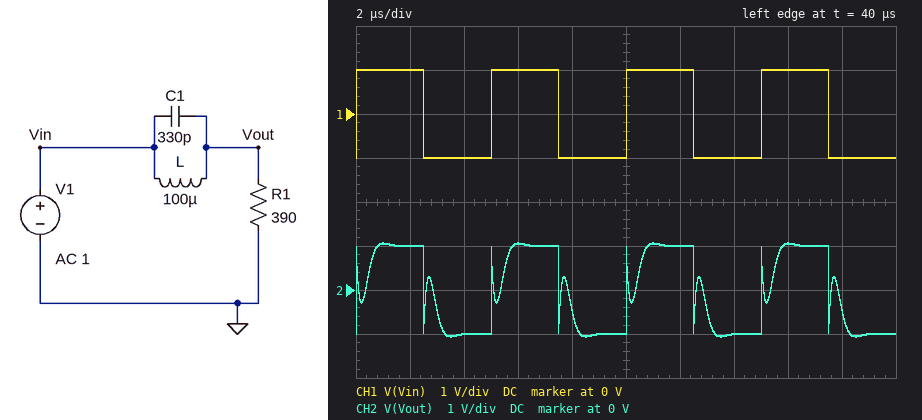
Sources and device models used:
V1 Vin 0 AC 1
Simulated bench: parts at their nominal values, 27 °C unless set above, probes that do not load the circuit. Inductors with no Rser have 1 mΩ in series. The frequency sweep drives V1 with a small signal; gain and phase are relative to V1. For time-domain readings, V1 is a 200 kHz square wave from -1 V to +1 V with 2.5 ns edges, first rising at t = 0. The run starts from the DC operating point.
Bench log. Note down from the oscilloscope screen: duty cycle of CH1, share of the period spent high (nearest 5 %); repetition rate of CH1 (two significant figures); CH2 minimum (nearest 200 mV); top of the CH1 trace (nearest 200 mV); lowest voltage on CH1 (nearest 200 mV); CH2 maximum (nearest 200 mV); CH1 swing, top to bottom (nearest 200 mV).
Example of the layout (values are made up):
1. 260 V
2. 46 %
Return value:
1. 50 %
2. 200 kHz
3. -1.0 V
4. 1.0 V
5. -1.0 V
6. 1.0 V
7. 2.0 V
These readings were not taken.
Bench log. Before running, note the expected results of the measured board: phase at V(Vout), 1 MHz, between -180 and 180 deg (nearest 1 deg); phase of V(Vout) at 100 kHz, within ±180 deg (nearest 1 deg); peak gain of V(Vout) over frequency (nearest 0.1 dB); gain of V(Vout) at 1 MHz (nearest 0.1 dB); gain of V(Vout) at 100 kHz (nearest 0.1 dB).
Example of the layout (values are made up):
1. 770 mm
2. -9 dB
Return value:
1. 79 deg
2. -9 deg
3. 0 dB
4. -14.7 dB
5. -0.1 dB
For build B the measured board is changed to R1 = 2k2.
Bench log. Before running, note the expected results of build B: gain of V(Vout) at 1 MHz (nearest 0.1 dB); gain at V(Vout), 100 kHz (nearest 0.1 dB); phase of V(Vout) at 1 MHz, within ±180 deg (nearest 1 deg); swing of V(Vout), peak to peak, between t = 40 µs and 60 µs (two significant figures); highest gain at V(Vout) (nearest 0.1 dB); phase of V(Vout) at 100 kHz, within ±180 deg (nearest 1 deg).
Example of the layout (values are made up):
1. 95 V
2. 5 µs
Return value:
1. -2.8 dB
2. 0 dB
3. 43 deg
4. 2.5 V
5. 0 dB
6. -2 deg
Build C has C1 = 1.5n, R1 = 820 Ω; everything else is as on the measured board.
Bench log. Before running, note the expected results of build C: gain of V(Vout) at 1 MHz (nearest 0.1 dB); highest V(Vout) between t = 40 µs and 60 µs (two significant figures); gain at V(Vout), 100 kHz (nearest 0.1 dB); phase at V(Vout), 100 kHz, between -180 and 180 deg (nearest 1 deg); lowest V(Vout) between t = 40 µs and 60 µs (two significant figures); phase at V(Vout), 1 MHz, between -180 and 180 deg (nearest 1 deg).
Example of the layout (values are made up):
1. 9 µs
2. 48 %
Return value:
1. -0.1 dB
2. 1.2 V
3. 0 dB
4. -5 deg
5. -1.2 V
6. 9 deg
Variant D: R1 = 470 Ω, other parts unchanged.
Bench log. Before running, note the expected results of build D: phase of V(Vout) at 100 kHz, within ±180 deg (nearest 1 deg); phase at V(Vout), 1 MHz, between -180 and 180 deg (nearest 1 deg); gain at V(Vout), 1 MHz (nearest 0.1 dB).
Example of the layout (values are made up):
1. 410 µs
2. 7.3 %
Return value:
1. -8 deg
2. 77 deg
3. -13.1 dB
